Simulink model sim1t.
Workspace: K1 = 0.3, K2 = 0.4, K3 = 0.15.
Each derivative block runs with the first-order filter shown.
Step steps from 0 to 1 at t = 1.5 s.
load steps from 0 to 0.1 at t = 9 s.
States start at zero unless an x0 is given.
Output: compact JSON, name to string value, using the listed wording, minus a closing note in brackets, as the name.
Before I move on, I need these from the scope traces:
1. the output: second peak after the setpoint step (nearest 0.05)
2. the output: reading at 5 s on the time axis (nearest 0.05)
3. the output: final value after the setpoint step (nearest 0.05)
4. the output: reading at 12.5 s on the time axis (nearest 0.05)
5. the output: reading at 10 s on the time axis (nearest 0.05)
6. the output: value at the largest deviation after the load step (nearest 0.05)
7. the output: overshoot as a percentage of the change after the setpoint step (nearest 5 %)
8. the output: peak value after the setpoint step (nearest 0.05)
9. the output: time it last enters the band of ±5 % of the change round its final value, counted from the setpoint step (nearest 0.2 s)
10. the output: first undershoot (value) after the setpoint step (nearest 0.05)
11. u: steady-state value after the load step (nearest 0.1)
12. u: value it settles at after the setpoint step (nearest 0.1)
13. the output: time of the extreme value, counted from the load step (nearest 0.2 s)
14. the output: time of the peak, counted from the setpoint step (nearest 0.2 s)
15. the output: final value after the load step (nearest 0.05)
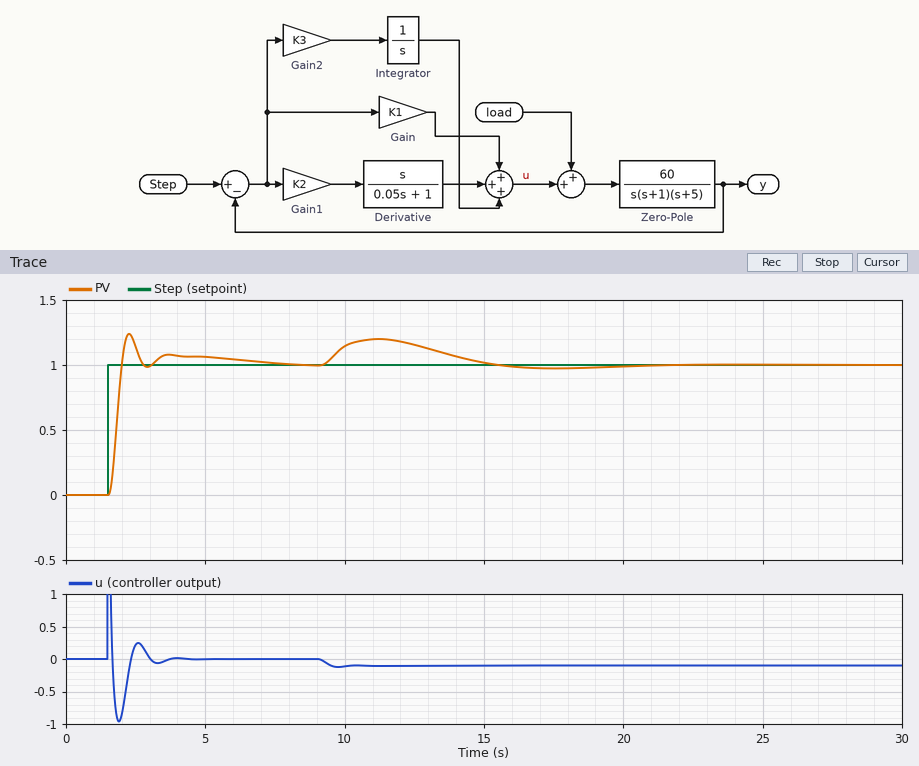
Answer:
{"the output: second peak after the setpoint step": "1.10", "the output: reading at 5 s on the time axis": "1.05", "the output: final value after the setpoint step": "1.00", "the output: reading at 12.5 s on the time axis": "1.15", "the output: reading at 10 s on the time axis": "1.15", "the output: value at the largest deviation after the load step": "1.20", "the output: overshoot as a percentage of the change after the setpoint step": "25 %", "the output: peak value after the setpoint step": "1.25", "the output: time it last enters the band of ±5 % of the change round its final value, counted from the setpoint step": "4.2 s", "the output: first undershoot (value) after the setpoint step": "1.00", "u: steady-state value after the load step": "-0.1", "u: value it settles at after the setpoint step": "0.0", "the output: time of the extreme value, counted from the load step": "2.2 s", "the output: time of the peak, counted from the setpoint step": "0.8 s", "the output: final value after the load step": "1.00"}
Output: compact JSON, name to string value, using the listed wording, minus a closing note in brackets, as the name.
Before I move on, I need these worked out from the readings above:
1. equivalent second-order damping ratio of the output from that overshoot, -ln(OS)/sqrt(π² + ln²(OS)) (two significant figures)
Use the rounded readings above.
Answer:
{"equivalent second-order damping ratio of the output from that overshoot, -ln(OS)/sqrt(π² + ln²(OS))": "0.40"}
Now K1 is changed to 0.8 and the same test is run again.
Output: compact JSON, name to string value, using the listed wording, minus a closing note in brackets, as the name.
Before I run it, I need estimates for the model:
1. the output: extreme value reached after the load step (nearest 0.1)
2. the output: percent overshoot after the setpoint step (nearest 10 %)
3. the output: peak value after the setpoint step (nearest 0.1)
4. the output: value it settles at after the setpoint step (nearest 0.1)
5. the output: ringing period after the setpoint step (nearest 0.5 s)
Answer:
{"the output: extreme value reached after the load step": "1.1", "the output: percent overshoot after the setpoint step": "50 %", "the output: peak value after the setpoint step": "1.5", "the output: value it settles at after the setpoint step": "1.0", "the output: ringing period after the setpoint step": "1.5 s"}
